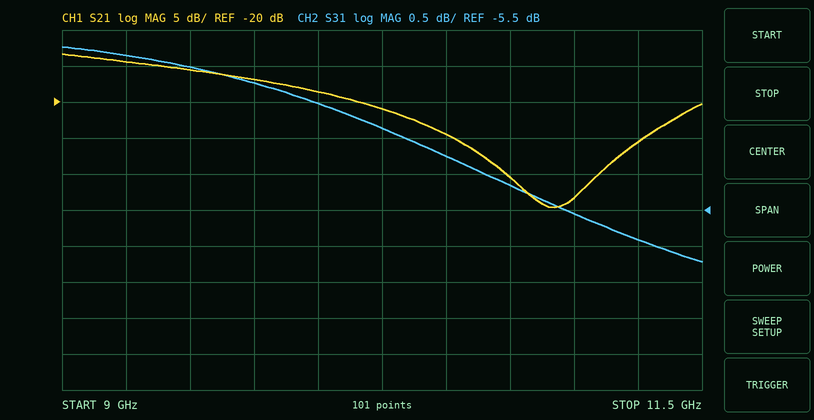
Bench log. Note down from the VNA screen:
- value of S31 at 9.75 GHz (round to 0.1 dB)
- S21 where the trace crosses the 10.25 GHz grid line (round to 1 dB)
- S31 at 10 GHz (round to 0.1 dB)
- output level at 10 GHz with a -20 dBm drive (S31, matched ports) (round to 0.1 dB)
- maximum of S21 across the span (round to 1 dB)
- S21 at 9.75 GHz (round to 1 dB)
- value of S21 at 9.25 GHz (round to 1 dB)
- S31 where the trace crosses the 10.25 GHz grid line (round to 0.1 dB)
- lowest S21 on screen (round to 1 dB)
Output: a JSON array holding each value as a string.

["-3.7 dB", "-21 dB", "-4.0 dB", "-24.0 dBm", "-13 dB", "-17 dB", "-14 dB", "-4.4 dB", "-35 dB"]
